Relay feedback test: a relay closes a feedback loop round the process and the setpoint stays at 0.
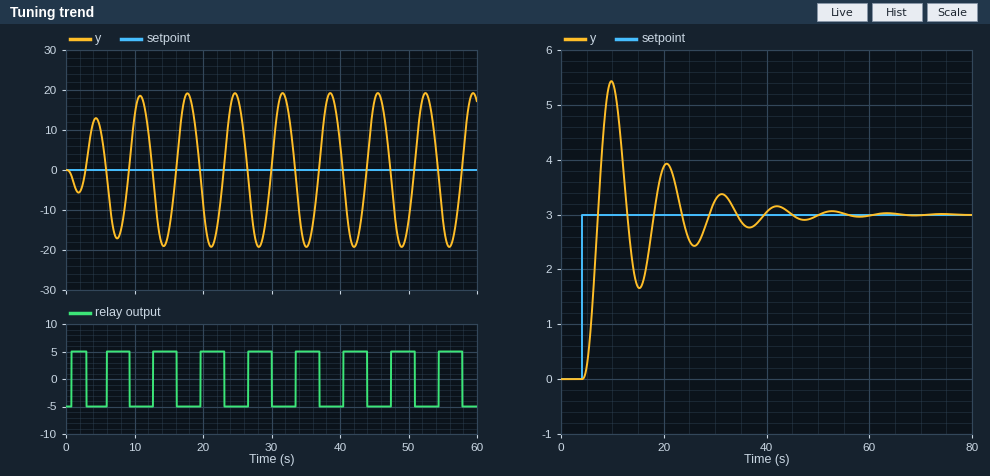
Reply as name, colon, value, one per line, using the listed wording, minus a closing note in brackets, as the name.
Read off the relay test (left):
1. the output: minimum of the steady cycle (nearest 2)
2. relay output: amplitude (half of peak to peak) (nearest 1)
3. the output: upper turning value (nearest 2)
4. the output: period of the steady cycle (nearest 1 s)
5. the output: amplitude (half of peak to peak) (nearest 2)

the output: minimum of the steady cycle: -20
relay output: amplitude (half of peak to peak): 5
the output: upper turning value: 20
the output: period of the steady cycle: 7 s
the output: amplitude (half of peak to peak): 20
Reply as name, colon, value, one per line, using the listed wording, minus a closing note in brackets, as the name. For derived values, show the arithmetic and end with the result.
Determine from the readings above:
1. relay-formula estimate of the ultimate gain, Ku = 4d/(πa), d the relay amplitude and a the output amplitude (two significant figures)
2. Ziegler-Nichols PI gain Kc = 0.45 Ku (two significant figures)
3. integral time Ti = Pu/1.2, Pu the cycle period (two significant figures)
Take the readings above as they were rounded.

relay-formula estimate of the ultimate gain, Ku = 4d/(πa), d the relay amplitude and a the output amplitude: 4 × 5 / (π × 20) = 0.32
Ziegler-Nichols PI gain Kc = 0.45 Ku: 0.45 × 0.32 = 0.14
integral time Ti = Pu/1.2, Pu the cycle period: 7 / 1.2 = 5.8 s
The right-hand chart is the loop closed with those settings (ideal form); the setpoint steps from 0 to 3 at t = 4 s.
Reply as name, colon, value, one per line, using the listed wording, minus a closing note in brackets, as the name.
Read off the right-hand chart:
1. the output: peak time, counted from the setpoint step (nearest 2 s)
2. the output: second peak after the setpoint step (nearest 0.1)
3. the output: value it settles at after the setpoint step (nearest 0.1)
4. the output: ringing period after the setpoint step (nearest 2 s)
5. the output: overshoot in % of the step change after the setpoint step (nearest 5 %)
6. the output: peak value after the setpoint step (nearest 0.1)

the output: peak time, counted from the setpoint step: 6 s
the output: second peak after the setpoint step: 3.9
the output: value it settles at after the setpoint step: 3.0
the output: ringing period after the setpoint step: 10 s
the output: overshoot in % of the step change after the setpoint step: 80 %
the output: peak value after the setpoint step: 5.4
